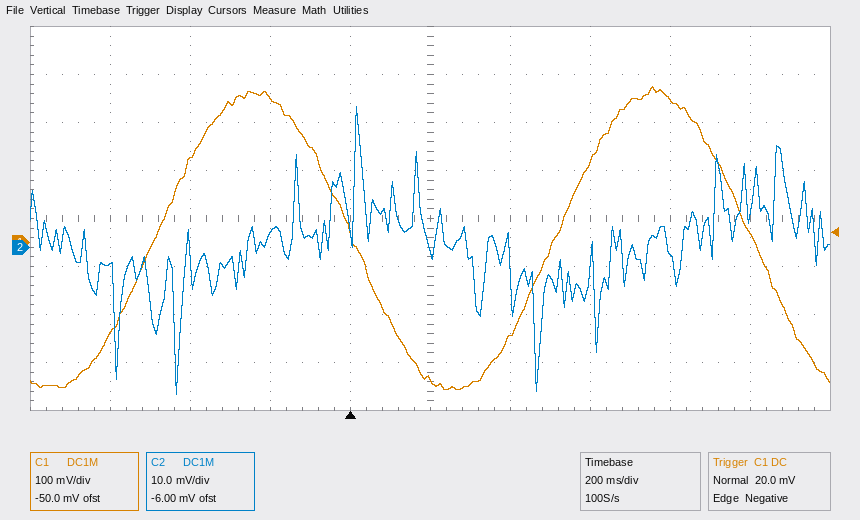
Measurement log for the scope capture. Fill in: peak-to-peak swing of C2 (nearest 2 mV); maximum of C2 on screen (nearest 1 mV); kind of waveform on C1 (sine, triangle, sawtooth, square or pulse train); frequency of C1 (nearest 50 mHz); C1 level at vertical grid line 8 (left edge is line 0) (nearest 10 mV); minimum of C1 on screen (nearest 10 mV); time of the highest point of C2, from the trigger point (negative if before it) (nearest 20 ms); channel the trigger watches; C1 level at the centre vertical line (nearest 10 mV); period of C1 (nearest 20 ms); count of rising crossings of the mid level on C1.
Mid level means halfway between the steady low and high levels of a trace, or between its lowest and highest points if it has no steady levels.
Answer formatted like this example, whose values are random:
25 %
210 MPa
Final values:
60 mV
29 mV
sine
1.00 Hz
300 mV
-310 mV
+20 ms
C1
-290 mV
1.00 s
2
